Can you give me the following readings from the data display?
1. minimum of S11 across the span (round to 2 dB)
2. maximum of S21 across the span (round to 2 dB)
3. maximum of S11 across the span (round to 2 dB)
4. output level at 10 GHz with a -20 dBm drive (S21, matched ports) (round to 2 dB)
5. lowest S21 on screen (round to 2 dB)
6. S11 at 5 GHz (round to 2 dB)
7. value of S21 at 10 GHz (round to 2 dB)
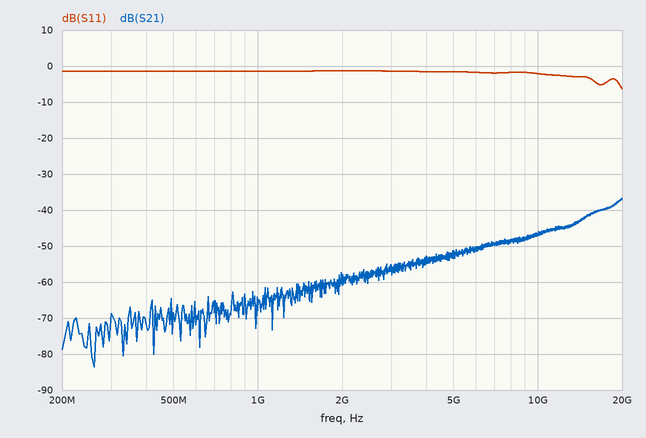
-6 dB
-36 dB
-2 dB
-66 dBm
-84 dB
-2 dB
-46 dB
